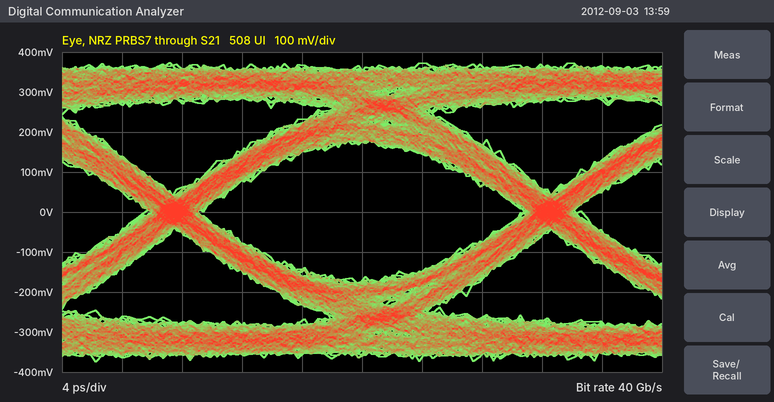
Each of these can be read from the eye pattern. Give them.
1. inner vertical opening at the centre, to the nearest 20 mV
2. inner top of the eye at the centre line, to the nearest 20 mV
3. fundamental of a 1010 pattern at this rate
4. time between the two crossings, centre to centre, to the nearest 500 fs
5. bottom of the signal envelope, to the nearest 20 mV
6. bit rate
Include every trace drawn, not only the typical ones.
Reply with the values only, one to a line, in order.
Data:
340 mV
180 mV
20 GHz
25.0 ps
-380 mV
40 Gb/s
